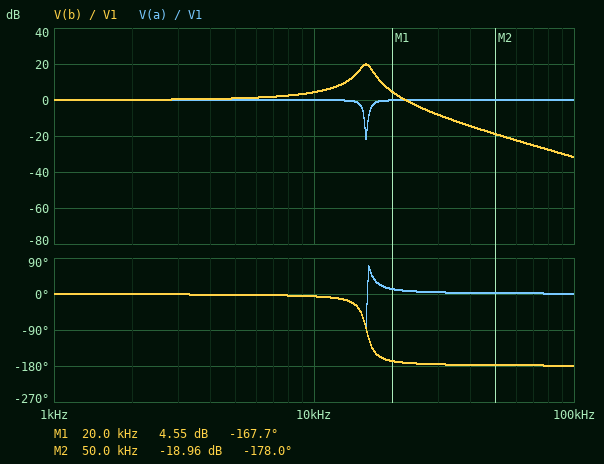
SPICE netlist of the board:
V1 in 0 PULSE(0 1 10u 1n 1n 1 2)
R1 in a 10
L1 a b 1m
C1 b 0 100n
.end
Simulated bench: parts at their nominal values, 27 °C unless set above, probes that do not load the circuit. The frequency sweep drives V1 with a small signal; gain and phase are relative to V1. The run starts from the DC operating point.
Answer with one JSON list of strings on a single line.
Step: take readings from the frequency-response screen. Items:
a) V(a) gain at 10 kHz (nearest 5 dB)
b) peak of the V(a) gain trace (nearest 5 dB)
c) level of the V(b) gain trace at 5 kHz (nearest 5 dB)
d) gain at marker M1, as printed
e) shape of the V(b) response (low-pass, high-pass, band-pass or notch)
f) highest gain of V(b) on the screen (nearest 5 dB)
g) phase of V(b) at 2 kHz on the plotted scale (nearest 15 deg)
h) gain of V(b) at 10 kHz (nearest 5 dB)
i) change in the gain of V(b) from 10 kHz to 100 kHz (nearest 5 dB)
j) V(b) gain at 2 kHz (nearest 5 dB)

["0 dB", "0 dB", "0 dB", "4.55 dB", "low-pass", "20 dB", "0 deg", "5 dB", "-35 dB", "0 dB"]
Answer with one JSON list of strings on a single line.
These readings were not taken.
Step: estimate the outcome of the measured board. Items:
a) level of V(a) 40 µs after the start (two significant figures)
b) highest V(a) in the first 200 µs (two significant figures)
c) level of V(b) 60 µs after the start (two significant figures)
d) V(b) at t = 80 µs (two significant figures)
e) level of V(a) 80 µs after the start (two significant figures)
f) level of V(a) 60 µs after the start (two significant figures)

["990 mV", "1.1 V", "820 mV", "440 mV", "950 mV", "1.1 V"]
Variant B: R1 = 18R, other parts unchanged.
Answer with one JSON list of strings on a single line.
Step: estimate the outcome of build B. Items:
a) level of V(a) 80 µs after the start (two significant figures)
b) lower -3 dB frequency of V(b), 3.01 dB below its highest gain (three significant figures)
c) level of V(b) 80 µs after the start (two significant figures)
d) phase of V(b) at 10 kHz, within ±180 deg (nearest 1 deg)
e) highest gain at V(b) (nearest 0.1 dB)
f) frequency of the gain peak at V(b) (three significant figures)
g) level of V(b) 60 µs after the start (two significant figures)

["940 mV", "14.3 kHz", "560 mV", "-11 deg", "14.9 dB", "15.8 kHz", "890 mV"]
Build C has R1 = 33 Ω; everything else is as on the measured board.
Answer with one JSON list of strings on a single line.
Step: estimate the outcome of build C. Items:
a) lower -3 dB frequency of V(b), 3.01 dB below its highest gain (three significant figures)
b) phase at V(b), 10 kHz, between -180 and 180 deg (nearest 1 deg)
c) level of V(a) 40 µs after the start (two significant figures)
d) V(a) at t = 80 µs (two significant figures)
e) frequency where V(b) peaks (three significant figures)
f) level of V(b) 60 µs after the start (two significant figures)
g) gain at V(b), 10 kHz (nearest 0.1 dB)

["12.5 kHz", "-19 deg", "960 mV", "940 mV", "15.5 kHz", "980 mV", "3.9 dB"]
